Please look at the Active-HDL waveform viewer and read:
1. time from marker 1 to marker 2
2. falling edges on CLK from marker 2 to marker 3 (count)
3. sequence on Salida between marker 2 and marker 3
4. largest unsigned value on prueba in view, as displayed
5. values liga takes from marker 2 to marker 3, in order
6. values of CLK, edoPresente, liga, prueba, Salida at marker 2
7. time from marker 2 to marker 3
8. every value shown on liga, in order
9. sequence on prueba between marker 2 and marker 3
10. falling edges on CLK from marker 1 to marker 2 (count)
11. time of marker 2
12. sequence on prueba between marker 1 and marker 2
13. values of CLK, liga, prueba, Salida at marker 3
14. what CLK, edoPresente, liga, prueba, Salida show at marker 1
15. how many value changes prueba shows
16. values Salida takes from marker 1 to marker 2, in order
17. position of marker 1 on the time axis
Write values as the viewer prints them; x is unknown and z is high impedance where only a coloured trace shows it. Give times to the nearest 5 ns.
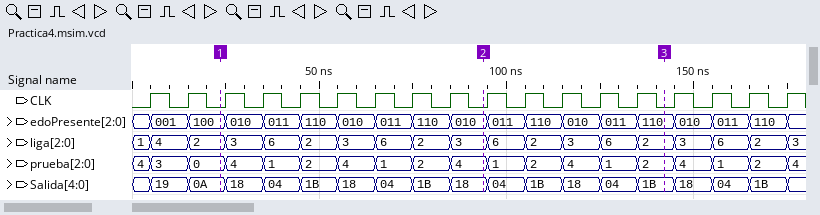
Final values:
70 ns
5
18, 04, 1B, 18, 04, 1B
4
3, 6, 2, 3, 6, 2
CLK=0, edoPresente=010, liga=3, prueba=4, Salida=18
50 ns
1, 4, 2, 3, 6, 2, 3, 6, 2, 3, 6, 2, 3, 6, 2, 3, 6, 2, 3
4, 1, 2, 4, 1, 2
7
95 ns
0, 4, 1, 2, 4, 1, 2, 4
CLK=0, liga=2, prueba=2, Salida=1B
CLK=0, edoPresente=100, liga=2, prueba=0, Salida=0A
18
0A, 18, 04, 1B, 18, 04, 1B, 18
25 ns
